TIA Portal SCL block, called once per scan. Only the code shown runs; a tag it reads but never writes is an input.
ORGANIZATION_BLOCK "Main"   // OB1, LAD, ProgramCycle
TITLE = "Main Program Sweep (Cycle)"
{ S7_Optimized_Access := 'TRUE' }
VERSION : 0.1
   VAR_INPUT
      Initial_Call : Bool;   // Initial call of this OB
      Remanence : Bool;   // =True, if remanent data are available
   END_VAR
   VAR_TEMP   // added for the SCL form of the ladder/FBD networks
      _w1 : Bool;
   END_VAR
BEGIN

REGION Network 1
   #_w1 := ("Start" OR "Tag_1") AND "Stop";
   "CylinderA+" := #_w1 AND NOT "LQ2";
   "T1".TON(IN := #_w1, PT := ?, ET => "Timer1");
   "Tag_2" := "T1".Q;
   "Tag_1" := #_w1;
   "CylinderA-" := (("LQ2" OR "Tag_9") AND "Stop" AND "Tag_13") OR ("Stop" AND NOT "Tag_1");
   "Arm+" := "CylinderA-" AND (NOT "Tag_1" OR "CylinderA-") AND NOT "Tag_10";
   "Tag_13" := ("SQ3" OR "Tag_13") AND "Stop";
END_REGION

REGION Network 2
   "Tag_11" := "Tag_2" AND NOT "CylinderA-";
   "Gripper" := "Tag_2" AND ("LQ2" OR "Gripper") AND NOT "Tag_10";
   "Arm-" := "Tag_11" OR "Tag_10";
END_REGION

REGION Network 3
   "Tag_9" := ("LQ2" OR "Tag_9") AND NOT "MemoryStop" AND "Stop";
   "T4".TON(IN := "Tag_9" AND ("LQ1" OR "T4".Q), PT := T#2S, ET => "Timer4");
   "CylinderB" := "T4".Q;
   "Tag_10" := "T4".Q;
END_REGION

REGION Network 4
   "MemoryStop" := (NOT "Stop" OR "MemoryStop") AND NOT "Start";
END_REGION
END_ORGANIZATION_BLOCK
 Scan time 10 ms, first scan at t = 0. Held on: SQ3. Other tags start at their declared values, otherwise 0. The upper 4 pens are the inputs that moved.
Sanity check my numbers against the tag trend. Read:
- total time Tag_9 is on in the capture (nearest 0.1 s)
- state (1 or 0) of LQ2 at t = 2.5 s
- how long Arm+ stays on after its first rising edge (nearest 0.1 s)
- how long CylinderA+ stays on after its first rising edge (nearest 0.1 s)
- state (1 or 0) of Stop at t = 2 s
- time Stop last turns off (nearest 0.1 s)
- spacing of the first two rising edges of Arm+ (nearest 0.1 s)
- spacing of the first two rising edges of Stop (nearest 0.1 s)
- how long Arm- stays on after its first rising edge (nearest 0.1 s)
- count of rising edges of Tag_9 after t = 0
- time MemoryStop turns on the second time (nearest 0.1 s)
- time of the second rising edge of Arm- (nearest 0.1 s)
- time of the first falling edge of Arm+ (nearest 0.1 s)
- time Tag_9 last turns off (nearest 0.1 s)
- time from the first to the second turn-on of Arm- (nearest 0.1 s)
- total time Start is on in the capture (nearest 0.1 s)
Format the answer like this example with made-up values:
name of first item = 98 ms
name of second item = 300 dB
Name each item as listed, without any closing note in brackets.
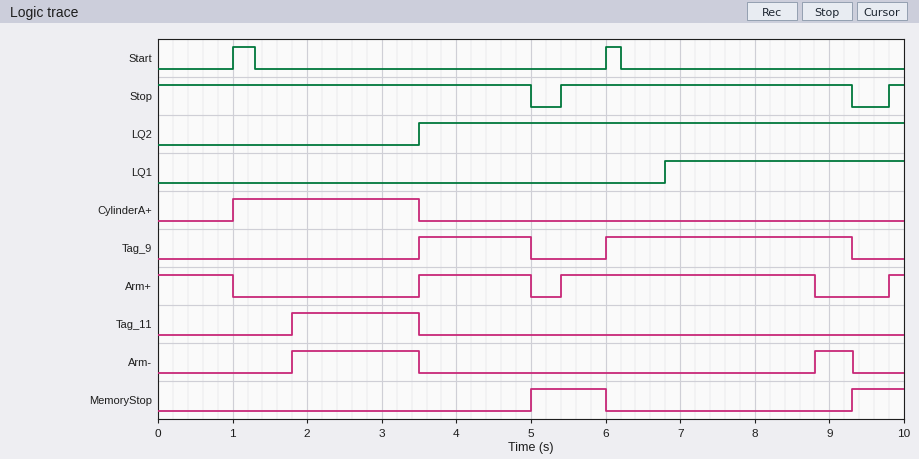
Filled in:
total time Tag_9 is on in the capture = 4.8 s
state (1 or 0) of LQ2 at t = 2.5 s = 0
how long Arm+ stays on after its first rising edge = 1.5 s
how long CylinderA+ stays on after its first rising edge = 2.5 s
state (1 or 0) of Stop at t = 2 s = 1
time Stop last turns off = 9.3 s
spacing of the first two rising edges of Arm+ = 1.9 s
spacing of the first two rising edges of Stop = 4.4 s
how long Arm- stays on after its first rising edge = 1.7 s
count of rising edges of Tag_9 after t = 0 = 2
time MemoryStop turns on the second time = 9.3 s
time of the second rising edge of Arm- = 8.8 s
time of the first falling edge of Arm+ = 1.0 s
time Tag_9 last turns off = 9.3 s
time from the first to the second turn-on of Arm- = 7.0 s
total time Start is on in the capture = 0.5 s
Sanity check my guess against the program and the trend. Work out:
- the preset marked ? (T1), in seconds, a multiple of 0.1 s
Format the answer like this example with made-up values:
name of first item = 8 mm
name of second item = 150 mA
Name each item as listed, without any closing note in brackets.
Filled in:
the preset marked ? (T1), in seconds, a multiple of 0.1 s = 0.8 s
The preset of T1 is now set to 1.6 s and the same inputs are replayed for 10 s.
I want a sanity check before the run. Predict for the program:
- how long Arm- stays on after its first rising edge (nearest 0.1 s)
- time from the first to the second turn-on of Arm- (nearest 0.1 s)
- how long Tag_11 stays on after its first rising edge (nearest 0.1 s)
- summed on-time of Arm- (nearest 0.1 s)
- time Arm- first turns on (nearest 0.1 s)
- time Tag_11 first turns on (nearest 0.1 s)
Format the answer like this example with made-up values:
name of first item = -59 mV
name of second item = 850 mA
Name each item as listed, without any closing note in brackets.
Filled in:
how long Arm- stays on after its first rising edge = 0.9 s
time from the first to the second turn-on of Arm- = 6.2 s
how long Tag_11 stays on after its first rising edge = 0.9 s
summed on-time of Arm- = 1.4 s
time Arm- first turns on = 2.6 s
time Tag_11 first turns on = 2.6 s
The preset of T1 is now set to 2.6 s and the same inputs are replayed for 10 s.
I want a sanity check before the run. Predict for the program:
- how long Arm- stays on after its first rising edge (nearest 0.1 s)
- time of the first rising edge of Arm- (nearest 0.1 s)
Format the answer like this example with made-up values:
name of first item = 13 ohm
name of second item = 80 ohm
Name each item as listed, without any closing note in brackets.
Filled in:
how long Arm- stays on after its first rising edge = 0.5 s
time of the first rising edge of Arm- = 8.8 s
